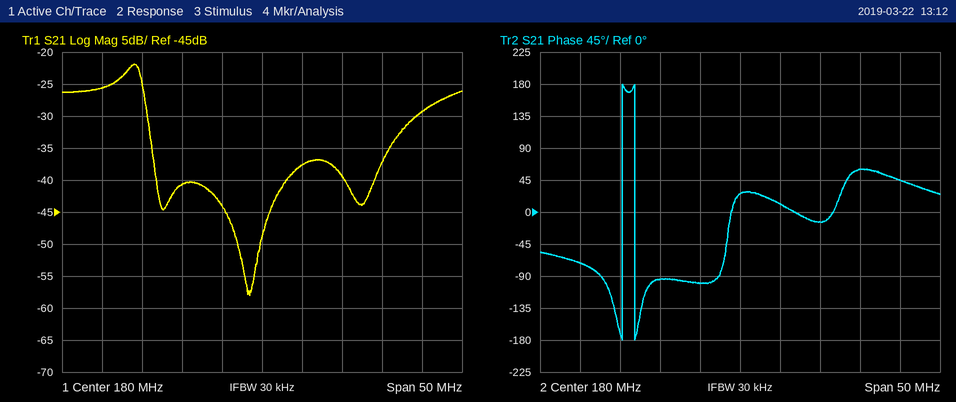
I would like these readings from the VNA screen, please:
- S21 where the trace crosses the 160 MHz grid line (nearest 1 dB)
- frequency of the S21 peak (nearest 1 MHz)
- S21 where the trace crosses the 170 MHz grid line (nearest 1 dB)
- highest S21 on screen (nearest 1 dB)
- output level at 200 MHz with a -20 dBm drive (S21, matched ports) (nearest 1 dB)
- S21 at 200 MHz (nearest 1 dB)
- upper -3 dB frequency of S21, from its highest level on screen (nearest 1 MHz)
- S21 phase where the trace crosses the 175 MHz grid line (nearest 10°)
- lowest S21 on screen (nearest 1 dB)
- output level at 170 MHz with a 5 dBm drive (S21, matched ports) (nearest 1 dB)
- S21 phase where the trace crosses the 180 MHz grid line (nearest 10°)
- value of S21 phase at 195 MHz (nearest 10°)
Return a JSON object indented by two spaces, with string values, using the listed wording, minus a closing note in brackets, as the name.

{
  "S21 where the trace crosses the 160 MHz grid line": "-26 dB",
  "frequency of the S21 peak": "164 MHz",
  "S21 where the trace crosses the 170 MHz grid line": "-41 dB",
  "highest S21 on screen": "-22 dB",
  "output level at 200 MHz with a -20 dBm drive (S21, matched ports)": "-49 dBm",
  "S21 at 200 MHz": "-29 dB",
  "upper -3 dB frequency of S21, from its highest level on screen": "165 MHz",
  "S21 phase where the trace crosses the 175 MHz grid line": "-100°",
  "lowest S21 on screen": "-58 dB",
  "output level at 170 MHz with a 5 dBm drive (S21, matched ports)": "-36 dBm",
  "S21 phase where the trace crosses the 180 MHz grid line": "30°",
  "value of S21 phase at 195 MHz": "60°"
}
